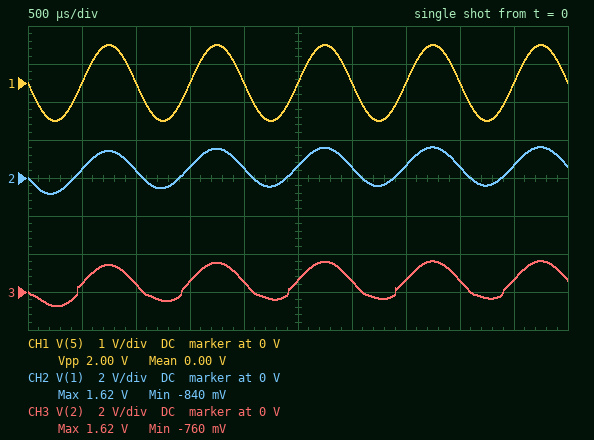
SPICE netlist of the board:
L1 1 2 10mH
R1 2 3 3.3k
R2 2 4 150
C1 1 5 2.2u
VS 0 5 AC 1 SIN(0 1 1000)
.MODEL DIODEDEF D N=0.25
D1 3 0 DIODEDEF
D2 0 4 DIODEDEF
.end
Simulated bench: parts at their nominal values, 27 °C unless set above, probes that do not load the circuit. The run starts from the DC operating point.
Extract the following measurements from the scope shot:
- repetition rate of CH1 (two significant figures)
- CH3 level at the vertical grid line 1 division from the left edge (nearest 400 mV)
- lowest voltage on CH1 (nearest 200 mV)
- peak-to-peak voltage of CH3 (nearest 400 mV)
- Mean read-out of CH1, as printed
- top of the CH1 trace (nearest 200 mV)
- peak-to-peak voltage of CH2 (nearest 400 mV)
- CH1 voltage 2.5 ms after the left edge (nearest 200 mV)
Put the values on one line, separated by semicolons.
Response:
1.0 kHz; 400 mV; -1.0 V; 2.4 V; 0.00 V; 1.0 V; 2.4 V; 0 V
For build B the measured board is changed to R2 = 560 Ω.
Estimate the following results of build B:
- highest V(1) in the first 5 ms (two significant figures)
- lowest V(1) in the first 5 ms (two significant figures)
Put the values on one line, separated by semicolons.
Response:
1.4 V; -920 mV
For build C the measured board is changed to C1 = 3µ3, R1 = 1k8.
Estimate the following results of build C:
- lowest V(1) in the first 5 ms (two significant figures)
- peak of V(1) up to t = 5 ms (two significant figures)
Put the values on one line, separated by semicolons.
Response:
-880 mV; 1.5 V
